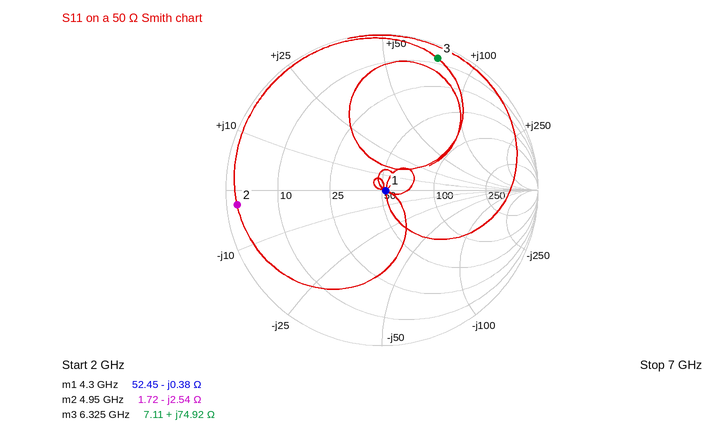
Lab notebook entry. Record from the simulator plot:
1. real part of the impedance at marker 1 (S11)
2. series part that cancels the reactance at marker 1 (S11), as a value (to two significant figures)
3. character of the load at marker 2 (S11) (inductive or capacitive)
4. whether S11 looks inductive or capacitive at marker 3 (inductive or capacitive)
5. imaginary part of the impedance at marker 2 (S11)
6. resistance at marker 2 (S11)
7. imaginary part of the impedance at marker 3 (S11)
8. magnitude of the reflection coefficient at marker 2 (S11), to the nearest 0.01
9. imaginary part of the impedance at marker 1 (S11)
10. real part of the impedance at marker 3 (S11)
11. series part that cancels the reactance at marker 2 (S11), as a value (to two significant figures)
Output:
52.45 Ω
14 pH
capacitive
inductive
-2.54 Ω
1.72 Ω
+74.92 Ω
0.93
-0.38 Ω
7.11 Ω
82 pH
